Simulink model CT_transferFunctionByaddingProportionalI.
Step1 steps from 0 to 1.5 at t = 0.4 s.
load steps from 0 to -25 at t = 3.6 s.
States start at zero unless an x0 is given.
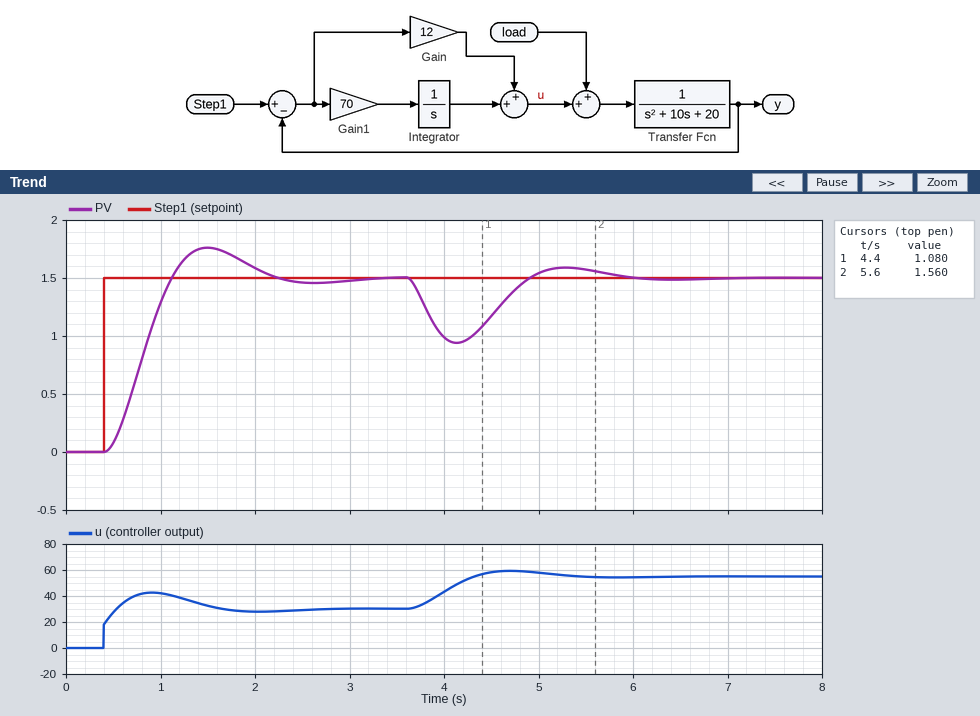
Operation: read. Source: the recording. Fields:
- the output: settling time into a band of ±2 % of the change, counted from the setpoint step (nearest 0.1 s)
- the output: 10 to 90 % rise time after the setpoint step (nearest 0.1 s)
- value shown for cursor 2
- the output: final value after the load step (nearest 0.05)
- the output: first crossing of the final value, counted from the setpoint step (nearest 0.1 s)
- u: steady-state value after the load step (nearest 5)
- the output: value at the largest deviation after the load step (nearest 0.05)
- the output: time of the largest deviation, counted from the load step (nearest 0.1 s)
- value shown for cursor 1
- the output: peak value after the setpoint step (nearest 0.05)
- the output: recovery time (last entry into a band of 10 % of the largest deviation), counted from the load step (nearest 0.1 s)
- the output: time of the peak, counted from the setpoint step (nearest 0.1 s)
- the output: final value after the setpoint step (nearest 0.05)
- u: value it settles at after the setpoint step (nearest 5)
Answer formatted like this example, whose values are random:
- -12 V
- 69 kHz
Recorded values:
- 2.5 s
- 0.5 s
- 1.560
- 1.50
- 0.7 s
- 55
- 0.95
- 0.5 s
- 1.080
- 1.75
- 2.0 s
- 1.1 s
- 1.50
- 30
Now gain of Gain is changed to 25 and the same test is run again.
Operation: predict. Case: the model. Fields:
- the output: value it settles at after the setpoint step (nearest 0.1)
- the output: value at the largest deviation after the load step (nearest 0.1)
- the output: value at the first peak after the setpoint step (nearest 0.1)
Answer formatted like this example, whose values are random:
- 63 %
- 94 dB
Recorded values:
- 1.5
- 1.0
- 1.6
